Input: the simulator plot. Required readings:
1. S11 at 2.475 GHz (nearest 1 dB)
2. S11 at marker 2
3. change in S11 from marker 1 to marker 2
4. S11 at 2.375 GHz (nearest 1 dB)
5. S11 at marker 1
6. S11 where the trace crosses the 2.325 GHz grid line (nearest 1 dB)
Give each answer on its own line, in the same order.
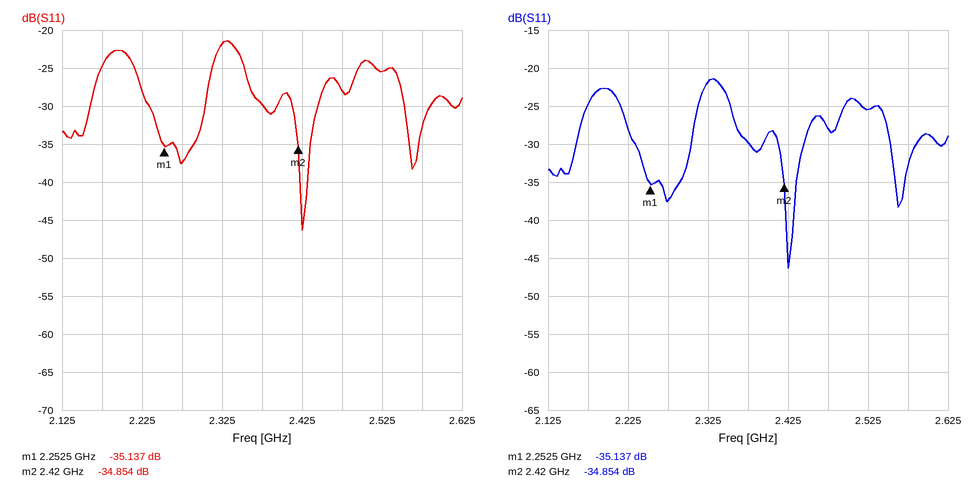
-28 dB
-34.854 dB
0.283 dB
-30 dB
-35.137 dB
-22 dB
